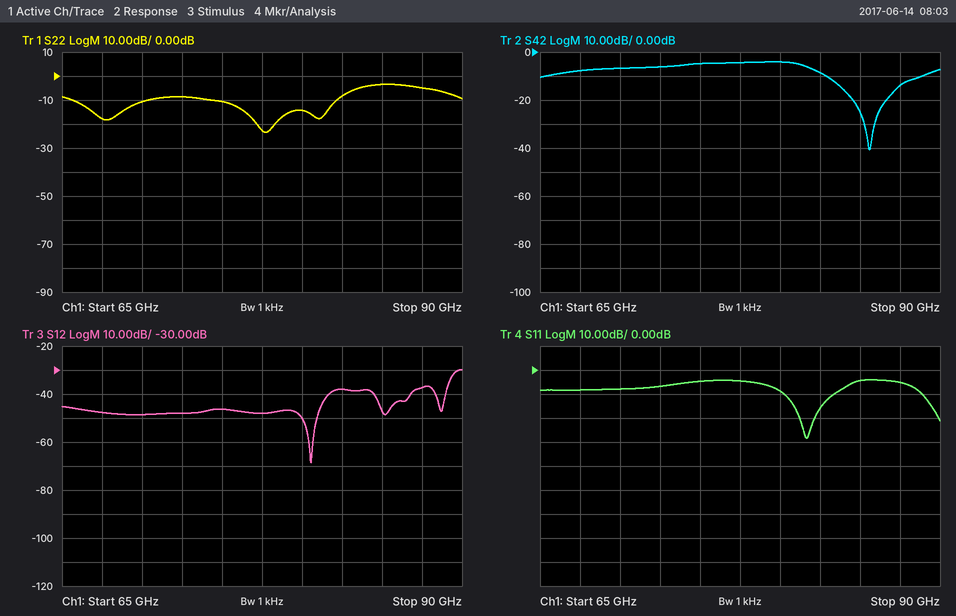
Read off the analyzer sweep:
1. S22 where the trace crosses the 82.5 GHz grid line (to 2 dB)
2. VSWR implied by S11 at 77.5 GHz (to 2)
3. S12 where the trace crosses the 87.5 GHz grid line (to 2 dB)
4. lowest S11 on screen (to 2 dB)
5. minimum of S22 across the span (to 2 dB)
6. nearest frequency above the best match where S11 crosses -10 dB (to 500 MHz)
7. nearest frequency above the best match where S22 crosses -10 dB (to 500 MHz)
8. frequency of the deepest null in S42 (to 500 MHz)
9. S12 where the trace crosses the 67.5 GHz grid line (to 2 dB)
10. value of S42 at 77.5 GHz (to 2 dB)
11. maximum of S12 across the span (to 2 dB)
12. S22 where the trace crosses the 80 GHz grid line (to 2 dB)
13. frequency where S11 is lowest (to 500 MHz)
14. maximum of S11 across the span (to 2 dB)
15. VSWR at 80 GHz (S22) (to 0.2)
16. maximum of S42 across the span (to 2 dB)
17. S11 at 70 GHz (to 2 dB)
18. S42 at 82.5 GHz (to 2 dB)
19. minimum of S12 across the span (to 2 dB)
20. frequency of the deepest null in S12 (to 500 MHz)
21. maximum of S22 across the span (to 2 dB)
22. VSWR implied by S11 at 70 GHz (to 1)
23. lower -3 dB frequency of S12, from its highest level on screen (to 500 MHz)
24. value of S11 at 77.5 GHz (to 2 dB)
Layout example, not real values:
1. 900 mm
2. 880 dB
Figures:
1. -8 dB
2. 4
3. -38 dB
4. -28 dB
5. -24 dB
6. 83.5 GHz
7. 82.0 GHz
8. 85.5 GHz
9. -48 dB
10. -4 dB
11. -30 dB
12. -14 dB
13. 81.5 GHz
14. -4 dB
15. 1.4
16. -4 dB
17. -8 dB
18. -8 dB
19. -68 dB
20. 80.5 GHz
21. -4 dB
22. 2
23. 89.5 GHz
24. -4 dB
